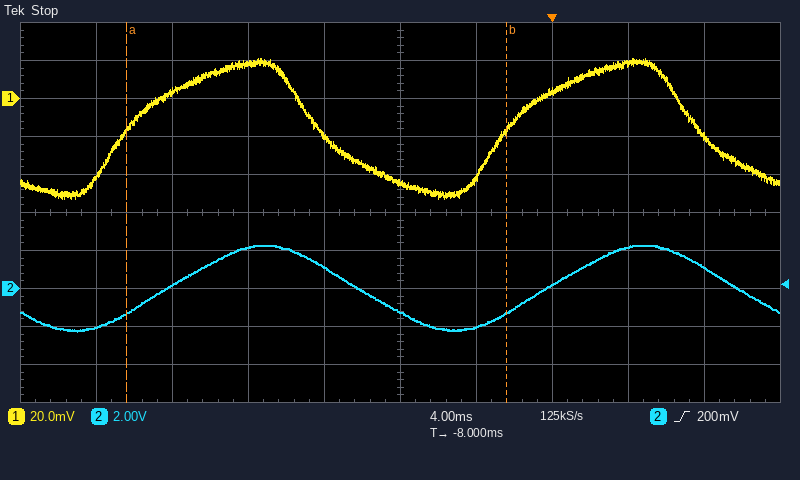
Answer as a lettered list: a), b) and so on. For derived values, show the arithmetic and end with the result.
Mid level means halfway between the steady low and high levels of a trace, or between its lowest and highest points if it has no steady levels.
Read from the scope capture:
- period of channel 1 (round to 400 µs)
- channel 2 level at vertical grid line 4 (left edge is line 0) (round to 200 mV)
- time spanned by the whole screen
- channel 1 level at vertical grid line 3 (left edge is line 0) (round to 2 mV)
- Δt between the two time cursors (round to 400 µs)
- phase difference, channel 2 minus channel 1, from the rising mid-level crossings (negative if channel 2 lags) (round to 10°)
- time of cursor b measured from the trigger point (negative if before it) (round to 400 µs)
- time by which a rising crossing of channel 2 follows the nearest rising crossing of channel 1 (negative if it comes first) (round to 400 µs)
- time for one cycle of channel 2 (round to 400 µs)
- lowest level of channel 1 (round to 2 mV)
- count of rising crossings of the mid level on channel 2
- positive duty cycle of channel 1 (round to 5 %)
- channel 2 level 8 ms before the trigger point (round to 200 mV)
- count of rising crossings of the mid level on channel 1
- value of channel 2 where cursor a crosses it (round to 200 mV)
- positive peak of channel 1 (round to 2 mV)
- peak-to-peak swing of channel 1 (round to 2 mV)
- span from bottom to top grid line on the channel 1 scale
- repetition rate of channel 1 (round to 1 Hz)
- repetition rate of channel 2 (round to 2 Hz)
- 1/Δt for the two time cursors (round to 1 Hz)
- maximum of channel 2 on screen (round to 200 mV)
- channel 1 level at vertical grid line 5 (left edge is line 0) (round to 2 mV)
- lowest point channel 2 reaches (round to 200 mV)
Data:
a) 20.0 ms
b) 1.2 V
c) 40 ms
d) 18 mV
e) 20.0 ms
f) −360° × (+2.0 ms) / 20.0 ms ≈ -36.0°, so -40° to the nearest 10°
g) -2.4 ms
h) +2.0 ms
i) 20.0 ms
j) -52 mV
k) 2
l) 50 %
m) -1.2 V
n) 2
o) -1.4 V
p) 22 mV
q) 22 mV − (-52 mV) = 74 mV
r) 200 mV
s) 1 / 20.0 ms ≈ 50 Hz
t) 1 / 20.0 ms ≈ 50 Hz
u) 1 / 20.0 ms ≈ 50 Hz
v) 2.2 V
w) -44 mV
x) -2.2 V
